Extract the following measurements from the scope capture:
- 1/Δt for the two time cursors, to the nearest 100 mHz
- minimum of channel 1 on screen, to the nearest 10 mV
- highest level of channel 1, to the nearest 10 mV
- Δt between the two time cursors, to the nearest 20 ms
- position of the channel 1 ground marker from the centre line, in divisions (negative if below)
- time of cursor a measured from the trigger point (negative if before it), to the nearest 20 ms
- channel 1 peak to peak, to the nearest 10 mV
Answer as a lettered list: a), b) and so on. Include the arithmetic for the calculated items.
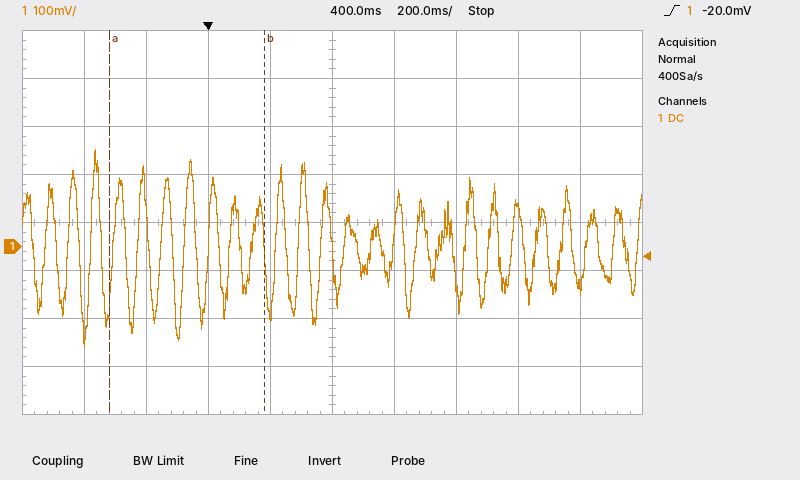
a) 1 / 500 ms ≈ 2.0 Hz
b) -210 mV
c) 200 mV
d) 500 ms
e) -0.5 div
f) -320 ms
g) 200 mV − (-210 mV) = 410 mV
